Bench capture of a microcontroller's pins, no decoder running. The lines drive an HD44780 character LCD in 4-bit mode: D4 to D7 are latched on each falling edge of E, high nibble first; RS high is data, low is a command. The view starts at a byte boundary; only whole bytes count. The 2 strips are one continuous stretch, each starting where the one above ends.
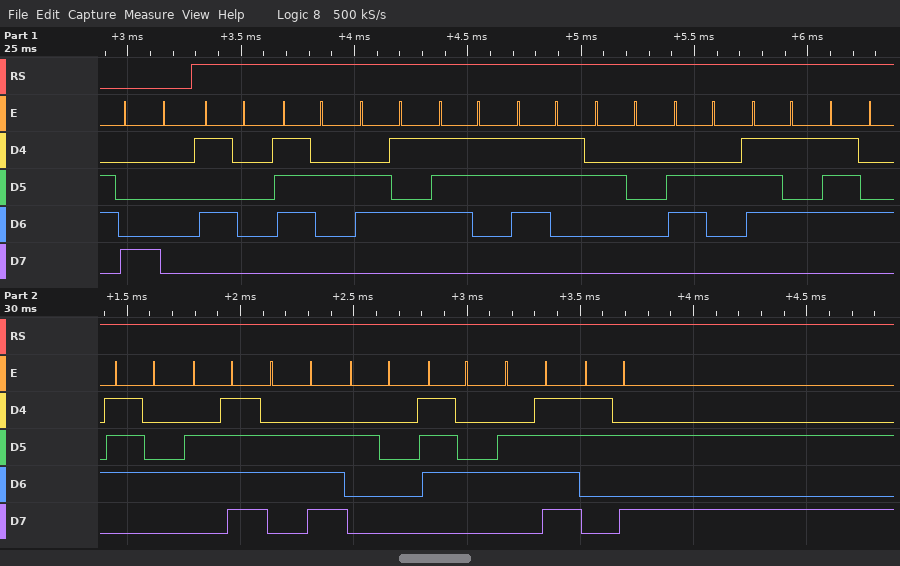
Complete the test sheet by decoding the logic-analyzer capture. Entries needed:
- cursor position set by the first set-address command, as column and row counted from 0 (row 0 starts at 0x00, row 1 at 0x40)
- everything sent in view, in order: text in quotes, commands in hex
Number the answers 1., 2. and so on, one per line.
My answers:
1. column 0, row 0
2. 0x80 "Press button to:"
